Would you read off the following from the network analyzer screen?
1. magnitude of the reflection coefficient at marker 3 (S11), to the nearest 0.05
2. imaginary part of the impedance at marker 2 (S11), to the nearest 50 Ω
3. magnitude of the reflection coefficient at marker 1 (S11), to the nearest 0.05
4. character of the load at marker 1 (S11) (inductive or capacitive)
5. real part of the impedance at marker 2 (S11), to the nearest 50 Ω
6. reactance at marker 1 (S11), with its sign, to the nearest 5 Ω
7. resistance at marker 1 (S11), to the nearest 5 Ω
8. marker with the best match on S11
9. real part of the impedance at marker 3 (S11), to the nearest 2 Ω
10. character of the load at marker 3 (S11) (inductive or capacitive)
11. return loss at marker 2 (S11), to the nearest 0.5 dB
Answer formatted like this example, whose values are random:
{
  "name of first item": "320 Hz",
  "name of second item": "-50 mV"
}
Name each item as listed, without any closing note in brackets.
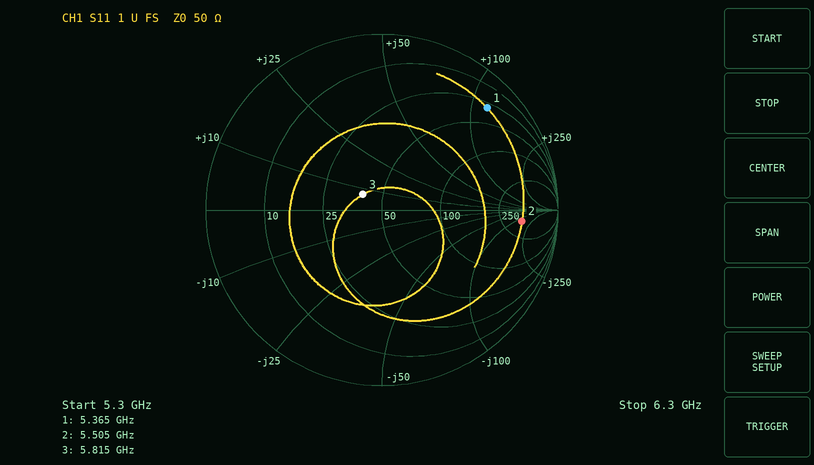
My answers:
{
  "magnitude of the reflection coefficient at marker 3 (S11), to the nearest 0.05": "0.15",
  "imaginary part of the impedance at marker 2 (S11), to the nearest 50 Ω": "-150 Ω",
  "magnitude of the reflection coefficient at marker 1 (S11), to the nearest 0.05": "0.85",
  "character of the load at marker 1 (S11)": "inductive",
  "real part of the impedance at marker 2 (S11), to the nearest 50 Ω": "400 Ω",
  "reactance at marker 1 (S11), with its sign, to the nearest 5 Ω": "+115 Ω",
  "resistance at marker 1 (S11), to the nearest 5 Ω": "30 Ω",
  "marker with the best match on S11": "marker 3",
  "real part of the impedance at marker 3 (S11), to the nearest 2 Ω": "40 Ω",
  "character of the load at marker 3 (S11)": "inductive",
  "return loss at marker 2 (S11), to the nearest 0.5 dB": "2.0 dB"
}
